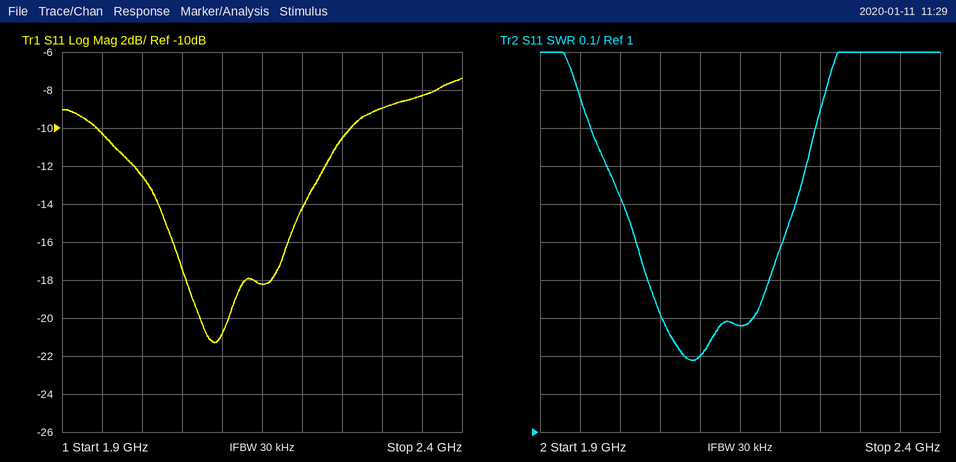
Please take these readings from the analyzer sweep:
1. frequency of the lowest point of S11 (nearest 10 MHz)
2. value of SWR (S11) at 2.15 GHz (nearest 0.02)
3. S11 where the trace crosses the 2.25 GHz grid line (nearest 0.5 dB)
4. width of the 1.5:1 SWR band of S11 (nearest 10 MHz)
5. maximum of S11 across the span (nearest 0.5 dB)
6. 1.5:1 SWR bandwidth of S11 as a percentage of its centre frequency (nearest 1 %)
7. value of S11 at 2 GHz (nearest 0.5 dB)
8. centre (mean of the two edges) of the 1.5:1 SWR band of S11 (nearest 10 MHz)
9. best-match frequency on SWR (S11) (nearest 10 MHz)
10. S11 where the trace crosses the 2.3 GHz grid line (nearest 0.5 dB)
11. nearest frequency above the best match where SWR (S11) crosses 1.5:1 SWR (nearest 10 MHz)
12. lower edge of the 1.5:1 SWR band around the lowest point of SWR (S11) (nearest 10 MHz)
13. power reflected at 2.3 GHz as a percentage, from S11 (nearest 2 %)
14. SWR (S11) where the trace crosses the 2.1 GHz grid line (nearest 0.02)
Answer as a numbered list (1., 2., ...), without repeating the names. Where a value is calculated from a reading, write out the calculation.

1. 2.09 GHz
2. 1.28
3. -10.5 dB
4. 2.20 GHz − 2.02 GHz = 180 MHz
5. -7.5 dB
6. 180 MHz / 2.11 GHz ≈ 9 %
7. -12.5 dB
8. 2.11 GHz
9. 2.09 GHz
10. -9.0 dB
11. 2.20 GHz
12. 2.02 GHz
13. 10^(-9/10) ≈ 12.6 %, so 12 % to the nearest 2 %
14. 1.20
